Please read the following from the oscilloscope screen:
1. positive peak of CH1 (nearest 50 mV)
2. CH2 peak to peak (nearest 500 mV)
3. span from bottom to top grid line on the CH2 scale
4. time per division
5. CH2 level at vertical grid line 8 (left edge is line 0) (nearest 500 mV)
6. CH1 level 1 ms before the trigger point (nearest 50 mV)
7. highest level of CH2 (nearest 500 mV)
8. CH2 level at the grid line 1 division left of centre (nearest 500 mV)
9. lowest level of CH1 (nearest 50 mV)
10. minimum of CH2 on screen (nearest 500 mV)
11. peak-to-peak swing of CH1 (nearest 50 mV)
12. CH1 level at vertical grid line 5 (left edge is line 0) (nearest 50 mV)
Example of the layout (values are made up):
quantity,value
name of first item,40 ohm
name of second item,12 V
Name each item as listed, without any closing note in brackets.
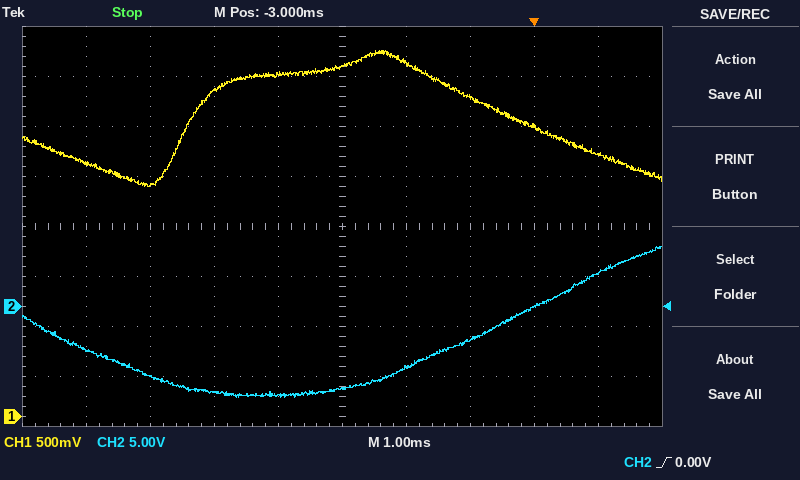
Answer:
quantity,value
positive peak of CH1,3.65 V
CH2 peak to peak,15.0 V
span from bottom to top grid line on the CH2 scale,40 V
time per division,1 ms
CH2 level at vertical grid line 8 (left edge is line 0),0.0 V
CH1 level 1 ms before the trigger point,3.20 V
highest level of CH2,6.0 V
CH2 level at the grid line 1 division left of centre,-9.0 V
lowest level of CH1,2.30 V
minimum of CH2 on screen,-9.0 V
peak-to-peak swing of CH1,1.35 V
CH1 level at vertical grid line 5 (left edge is line 0),3.50 V
